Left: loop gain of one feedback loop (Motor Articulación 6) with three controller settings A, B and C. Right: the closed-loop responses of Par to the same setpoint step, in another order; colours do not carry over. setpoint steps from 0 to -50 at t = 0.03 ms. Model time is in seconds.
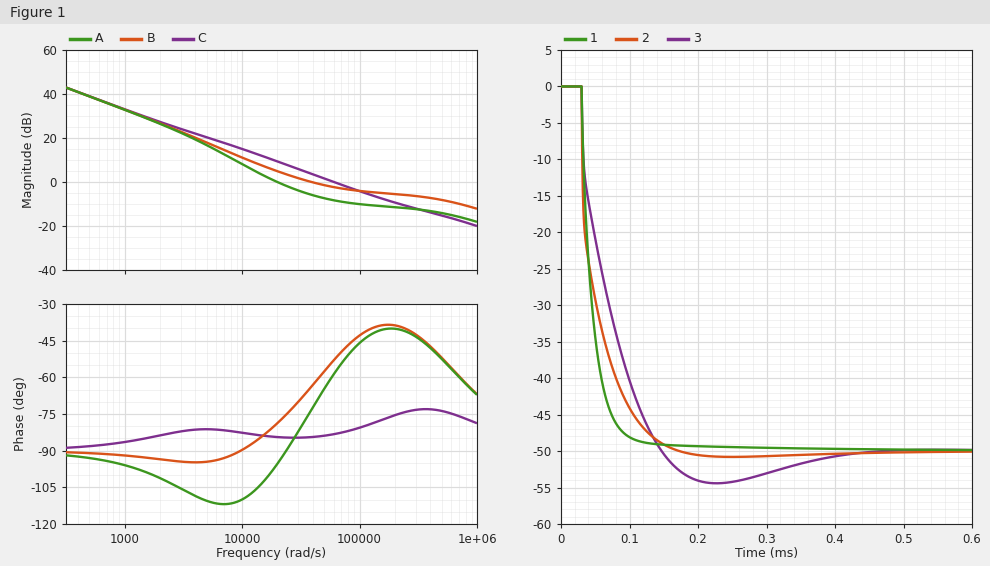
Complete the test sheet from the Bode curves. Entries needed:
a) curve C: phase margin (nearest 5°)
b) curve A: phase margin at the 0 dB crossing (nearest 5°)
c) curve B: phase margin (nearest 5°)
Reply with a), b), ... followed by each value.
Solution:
a) 95°
b) 85°
c) 115°
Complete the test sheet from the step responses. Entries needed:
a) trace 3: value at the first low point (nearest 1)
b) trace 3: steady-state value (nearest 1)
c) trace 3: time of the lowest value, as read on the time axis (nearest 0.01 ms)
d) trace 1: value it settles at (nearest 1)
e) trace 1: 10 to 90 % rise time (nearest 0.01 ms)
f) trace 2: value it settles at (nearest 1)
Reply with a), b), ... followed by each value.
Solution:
a) -54
b) -50
c) 0.23 ms
d) -50
e) 0.04 ms
f) -50
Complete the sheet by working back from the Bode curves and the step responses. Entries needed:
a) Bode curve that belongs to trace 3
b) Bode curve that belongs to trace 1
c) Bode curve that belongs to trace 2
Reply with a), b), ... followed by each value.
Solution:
a) A
b) C
c) B
